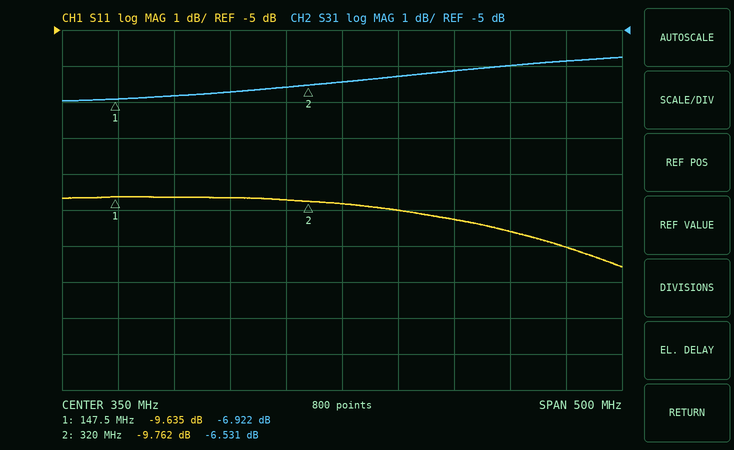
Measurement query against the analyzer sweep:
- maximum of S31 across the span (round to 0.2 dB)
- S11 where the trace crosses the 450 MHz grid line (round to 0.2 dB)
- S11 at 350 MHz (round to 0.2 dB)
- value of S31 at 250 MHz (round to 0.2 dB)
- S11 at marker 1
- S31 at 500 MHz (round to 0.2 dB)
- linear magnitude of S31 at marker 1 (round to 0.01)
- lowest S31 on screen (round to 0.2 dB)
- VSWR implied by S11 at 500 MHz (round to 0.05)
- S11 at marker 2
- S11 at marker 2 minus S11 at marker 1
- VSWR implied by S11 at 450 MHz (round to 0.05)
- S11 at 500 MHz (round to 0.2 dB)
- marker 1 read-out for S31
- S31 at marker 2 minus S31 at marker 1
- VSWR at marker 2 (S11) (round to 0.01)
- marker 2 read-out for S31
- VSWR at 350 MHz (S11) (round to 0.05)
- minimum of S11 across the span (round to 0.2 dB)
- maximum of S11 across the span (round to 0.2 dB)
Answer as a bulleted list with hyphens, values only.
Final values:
- -5.8 dB
- -10.2 dB
- -9.8 dB
- -6.8 dB
- -9.635 dB
- -6.0 dB
- 0.45
- -7.0 dB
- 1.85
- -9.762 dB
- -0.127 dB
- 1.90
- -10.6 dB
- -6.922 dB
- 0.391 dB
- 1.96
- -6.531 dB
- 1.95
- -11.6 dB
- -9.6 dB
